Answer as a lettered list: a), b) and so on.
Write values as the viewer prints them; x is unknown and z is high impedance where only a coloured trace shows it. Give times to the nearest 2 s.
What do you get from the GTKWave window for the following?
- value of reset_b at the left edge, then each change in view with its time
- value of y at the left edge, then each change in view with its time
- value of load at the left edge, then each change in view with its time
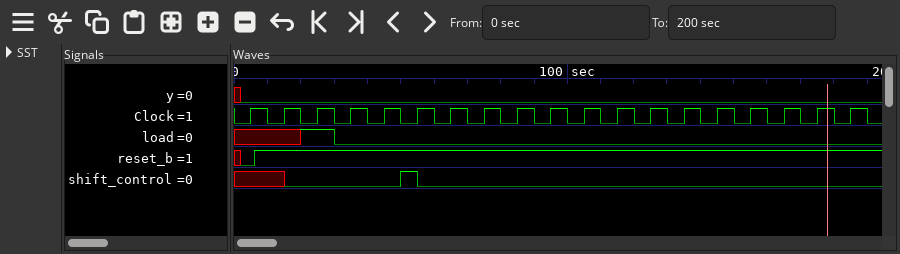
a) x, 0 at 2 s, 1 at 6 s
b) x, 0 at 2 s
c) x, 1 at 20 s, 0 at 30 s
